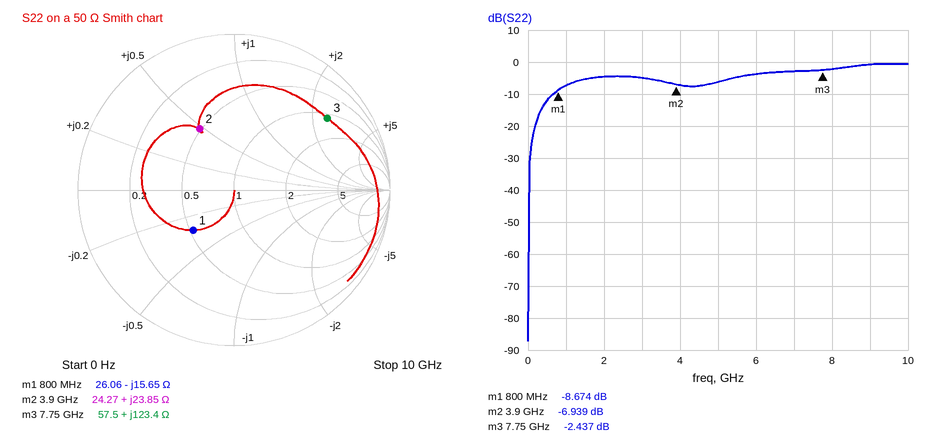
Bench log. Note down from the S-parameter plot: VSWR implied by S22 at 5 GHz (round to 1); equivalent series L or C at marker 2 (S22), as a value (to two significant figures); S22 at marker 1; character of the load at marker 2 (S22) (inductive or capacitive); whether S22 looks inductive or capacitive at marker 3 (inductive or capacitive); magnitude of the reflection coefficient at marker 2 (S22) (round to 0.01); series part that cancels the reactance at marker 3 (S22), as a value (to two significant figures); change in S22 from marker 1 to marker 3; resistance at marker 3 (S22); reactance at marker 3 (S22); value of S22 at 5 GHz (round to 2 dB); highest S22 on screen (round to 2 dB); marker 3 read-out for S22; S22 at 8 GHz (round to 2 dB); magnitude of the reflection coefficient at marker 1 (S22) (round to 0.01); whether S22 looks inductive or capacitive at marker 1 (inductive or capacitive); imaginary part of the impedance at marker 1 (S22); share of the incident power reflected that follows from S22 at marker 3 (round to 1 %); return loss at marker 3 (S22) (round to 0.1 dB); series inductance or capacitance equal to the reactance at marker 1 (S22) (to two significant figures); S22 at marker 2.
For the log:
3
970 pH
-8.674 dB
inductive
inductive
0.45
170 fF
6.237 dB
57.5 Ω
+123.4 Ω
-6 dB
0 dB
-2.437 dB
-2 dB
0.37
capacitive
-15.65 Ω
57 %
2.4 dB
13 pF
-6.939 dB
